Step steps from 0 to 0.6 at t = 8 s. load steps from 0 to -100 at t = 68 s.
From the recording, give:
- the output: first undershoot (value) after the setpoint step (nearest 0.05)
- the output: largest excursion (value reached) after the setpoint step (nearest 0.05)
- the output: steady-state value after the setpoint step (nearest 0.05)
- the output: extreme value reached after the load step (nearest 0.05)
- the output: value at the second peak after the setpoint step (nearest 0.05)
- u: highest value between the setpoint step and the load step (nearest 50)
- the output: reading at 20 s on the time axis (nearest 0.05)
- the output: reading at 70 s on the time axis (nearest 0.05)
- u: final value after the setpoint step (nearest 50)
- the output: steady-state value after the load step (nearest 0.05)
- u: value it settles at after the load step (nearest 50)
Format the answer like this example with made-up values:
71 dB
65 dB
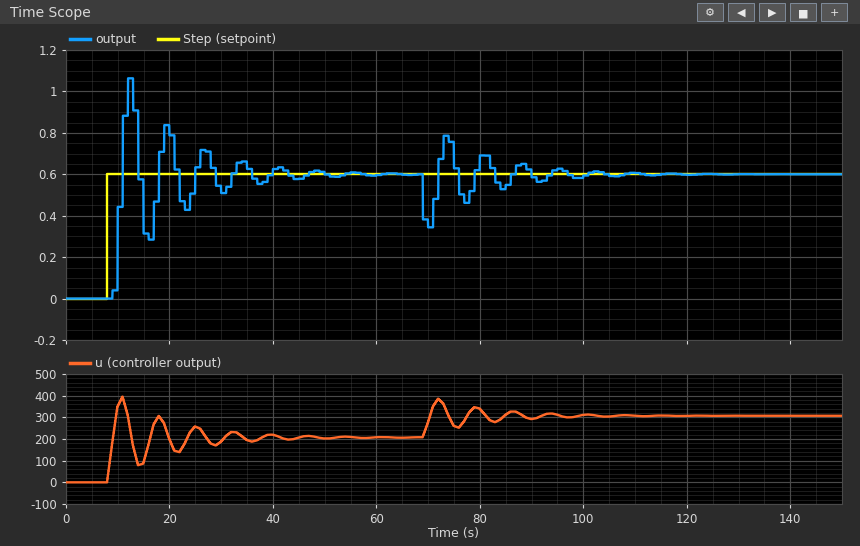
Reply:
0.30
1.05
0.60
0.35
0.85
400
0.80
0.35
200
0.60
300
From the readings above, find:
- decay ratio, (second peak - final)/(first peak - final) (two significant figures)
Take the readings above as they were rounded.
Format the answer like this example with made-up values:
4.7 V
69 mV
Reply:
0.56
